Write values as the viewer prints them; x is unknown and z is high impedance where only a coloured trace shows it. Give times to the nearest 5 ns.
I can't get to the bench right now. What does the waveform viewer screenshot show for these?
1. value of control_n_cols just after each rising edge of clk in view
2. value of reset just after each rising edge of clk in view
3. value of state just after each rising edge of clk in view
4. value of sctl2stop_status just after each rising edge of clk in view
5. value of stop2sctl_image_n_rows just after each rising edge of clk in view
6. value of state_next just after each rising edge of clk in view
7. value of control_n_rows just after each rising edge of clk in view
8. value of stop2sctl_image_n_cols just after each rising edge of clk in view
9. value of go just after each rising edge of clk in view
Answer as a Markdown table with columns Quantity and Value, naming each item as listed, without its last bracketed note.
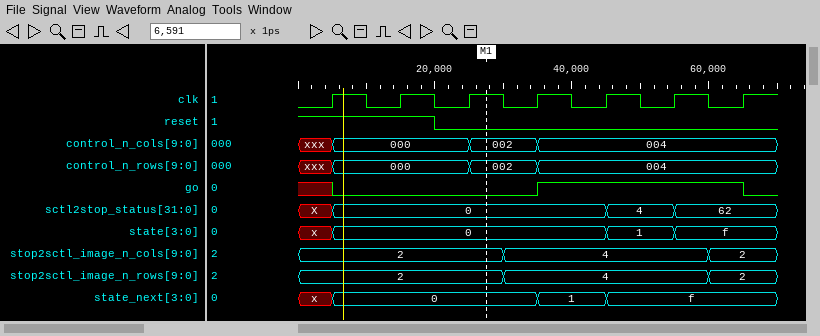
| Quantity | Value |
|---|---|
| value of control_n_cols just after each rising edge of clk in view | 000, 000, 002, 004, 004, 004, 004 |
| value of reset just after each rising edge of clk in view | 1 1 0 0 0 0 0 |
| value of state just after each rising edge of clk in view | 0, 0, 0, 0, 1, f, f |
| value of sctl2stop_status just after each rising edge of clk in view | 0, 0, 0, 0, 4, 62, 62 |
| value of stop2sctl_image_n_rows just after each rising edge of clk in view | 2, 2, 2, 4, 4, 4, 2 |
| value of state_next just after each rising edge of clk in view | 0, 0, 0, 1, f, f, f |
| value of control_n_rows just after each rising edge of clk in view | 000, 000, 002, 004, 004, 004, 004 |
| value of stop2sctl_image_n_cols just after each rising edge of clk in view | 2, 2, 2, 4, 4, 4, 2 |
| value of go just after each rising edge of clk in view | 0 0 0 1 1 1 0 |
